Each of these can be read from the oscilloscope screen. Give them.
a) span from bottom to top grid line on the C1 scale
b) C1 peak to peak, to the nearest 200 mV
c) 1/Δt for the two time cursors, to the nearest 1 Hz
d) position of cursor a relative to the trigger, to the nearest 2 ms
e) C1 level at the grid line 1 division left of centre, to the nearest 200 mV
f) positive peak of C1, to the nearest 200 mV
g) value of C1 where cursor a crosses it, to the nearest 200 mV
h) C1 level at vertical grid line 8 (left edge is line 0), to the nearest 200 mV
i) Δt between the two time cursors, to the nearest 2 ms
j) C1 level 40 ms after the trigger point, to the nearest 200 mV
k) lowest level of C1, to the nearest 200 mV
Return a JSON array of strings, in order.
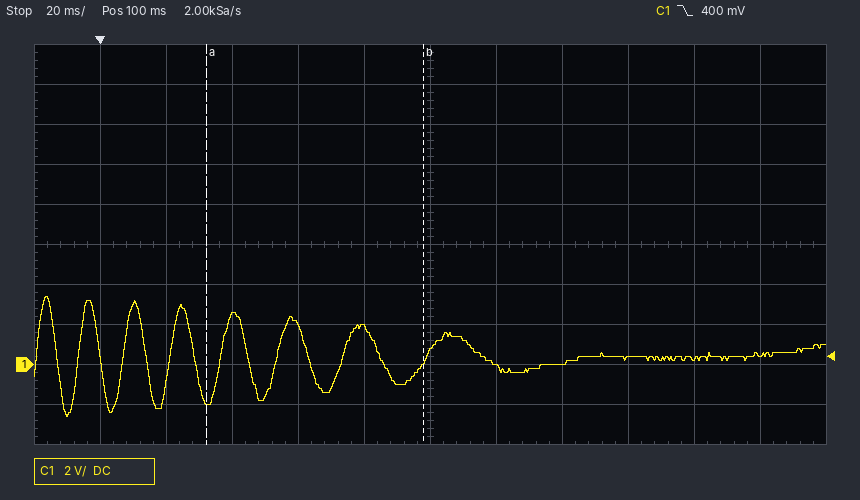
["20 V", "6.0 V", "15 Hz", "+32 ms", "1.8 V", "3.4 V", "-1.8 V", "0.0 V", "66 ms", "2.4 V", "-2.6 V"]
